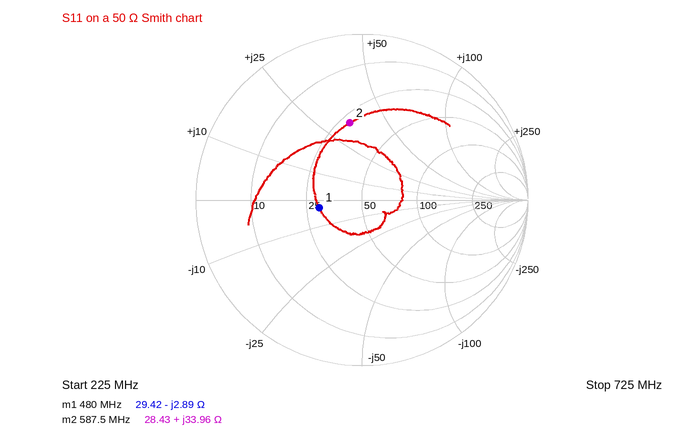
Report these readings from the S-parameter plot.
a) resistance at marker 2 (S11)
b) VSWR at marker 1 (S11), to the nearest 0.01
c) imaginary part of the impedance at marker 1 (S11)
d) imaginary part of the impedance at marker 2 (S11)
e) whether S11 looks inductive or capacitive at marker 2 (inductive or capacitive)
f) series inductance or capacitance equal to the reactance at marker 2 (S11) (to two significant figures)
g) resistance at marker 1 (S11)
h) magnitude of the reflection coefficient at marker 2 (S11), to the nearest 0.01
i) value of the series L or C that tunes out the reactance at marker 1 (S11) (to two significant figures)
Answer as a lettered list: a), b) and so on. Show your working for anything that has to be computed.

a) 28.43 Ω
b) 1.71
c) -2.89 Ω
d) +33.96 Ω
e) inductive
f) L = 33.96 Ω/(2π × 587.5 MHz) ≈ 9.2 nH
g) 29.42 Ω
h) 0.47
i) L = 2.89 Ω/(2π × 480 MHz) ≈ 958 pH, so 960 pH to two significant figures
